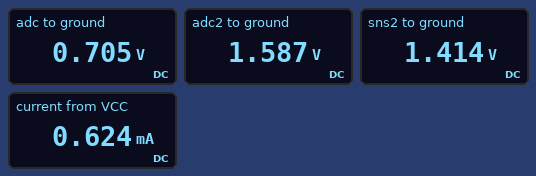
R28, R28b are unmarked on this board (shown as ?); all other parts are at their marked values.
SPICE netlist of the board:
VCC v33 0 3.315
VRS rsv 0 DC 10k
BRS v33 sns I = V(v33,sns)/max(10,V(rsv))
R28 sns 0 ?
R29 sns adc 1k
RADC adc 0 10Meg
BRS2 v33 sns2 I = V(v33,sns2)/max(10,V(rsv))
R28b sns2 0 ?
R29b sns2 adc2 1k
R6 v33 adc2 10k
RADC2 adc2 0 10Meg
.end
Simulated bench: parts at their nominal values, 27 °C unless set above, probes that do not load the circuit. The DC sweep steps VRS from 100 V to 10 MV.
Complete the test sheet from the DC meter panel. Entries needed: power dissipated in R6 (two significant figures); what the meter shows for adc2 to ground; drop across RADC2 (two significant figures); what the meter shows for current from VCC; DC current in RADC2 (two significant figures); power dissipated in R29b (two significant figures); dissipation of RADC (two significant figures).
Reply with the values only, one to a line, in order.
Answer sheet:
300 µW
1.587 V
1.6 V
0.624 mA
160 nA
30 µW
50 nW
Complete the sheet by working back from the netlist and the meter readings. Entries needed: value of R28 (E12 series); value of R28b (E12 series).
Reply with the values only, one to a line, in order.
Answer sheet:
2.7 kΩ
3.9 kΩ
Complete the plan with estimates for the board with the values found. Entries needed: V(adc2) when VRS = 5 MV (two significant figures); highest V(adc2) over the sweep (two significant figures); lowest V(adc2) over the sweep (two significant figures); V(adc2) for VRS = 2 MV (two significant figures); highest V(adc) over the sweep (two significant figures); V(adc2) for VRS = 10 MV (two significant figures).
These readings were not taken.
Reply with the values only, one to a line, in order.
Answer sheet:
1.1 V
3.2 V
1.1 V
1.1 V
3.2 V
1.1 V
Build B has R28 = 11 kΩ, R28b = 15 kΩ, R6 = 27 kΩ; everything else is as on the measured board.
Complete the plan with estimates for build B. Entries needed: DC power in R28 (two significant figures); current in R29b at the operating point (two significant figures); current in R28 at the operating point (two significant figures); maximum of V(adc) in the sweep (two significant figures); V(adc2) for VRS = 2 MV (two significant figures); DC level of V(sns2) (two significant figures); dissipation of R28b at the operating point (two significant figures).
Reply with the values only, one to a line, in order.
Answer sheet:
270 µW
39 µA
160 µA
3.3 V
1.2 V
2.2 V
330 µW
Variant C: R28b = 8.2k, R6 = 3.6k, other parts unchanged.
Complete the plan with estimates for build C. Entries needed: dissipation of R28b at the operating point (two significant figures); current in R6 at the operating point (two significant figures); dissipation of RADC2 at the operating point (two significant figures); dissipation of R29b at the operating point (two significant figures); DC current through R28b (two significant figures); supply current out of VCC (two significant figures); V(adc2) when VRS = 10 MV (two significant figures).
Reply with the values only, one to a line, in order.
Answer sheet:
700 µW
200 µA
670 nW
40 µW
290 µA
550 µA
2.4 V
